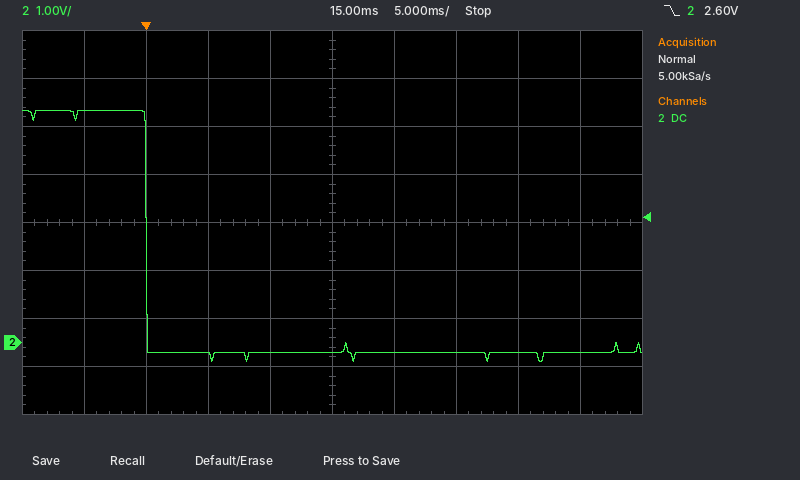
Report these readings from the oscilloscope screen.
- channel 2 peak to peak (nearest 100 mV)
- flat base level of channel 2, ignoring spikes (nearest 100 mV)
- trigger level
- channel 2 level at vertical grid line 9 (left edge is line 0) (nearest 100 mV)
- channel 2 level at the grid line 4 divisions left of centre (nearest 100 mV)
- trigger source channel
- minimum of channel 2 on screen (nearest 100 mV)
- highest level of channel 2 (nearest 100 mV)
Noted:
5.2 V
-200 mV
2.60 V
-200 mV
4.8 V
channel 2
-400 mV
4.8 V
